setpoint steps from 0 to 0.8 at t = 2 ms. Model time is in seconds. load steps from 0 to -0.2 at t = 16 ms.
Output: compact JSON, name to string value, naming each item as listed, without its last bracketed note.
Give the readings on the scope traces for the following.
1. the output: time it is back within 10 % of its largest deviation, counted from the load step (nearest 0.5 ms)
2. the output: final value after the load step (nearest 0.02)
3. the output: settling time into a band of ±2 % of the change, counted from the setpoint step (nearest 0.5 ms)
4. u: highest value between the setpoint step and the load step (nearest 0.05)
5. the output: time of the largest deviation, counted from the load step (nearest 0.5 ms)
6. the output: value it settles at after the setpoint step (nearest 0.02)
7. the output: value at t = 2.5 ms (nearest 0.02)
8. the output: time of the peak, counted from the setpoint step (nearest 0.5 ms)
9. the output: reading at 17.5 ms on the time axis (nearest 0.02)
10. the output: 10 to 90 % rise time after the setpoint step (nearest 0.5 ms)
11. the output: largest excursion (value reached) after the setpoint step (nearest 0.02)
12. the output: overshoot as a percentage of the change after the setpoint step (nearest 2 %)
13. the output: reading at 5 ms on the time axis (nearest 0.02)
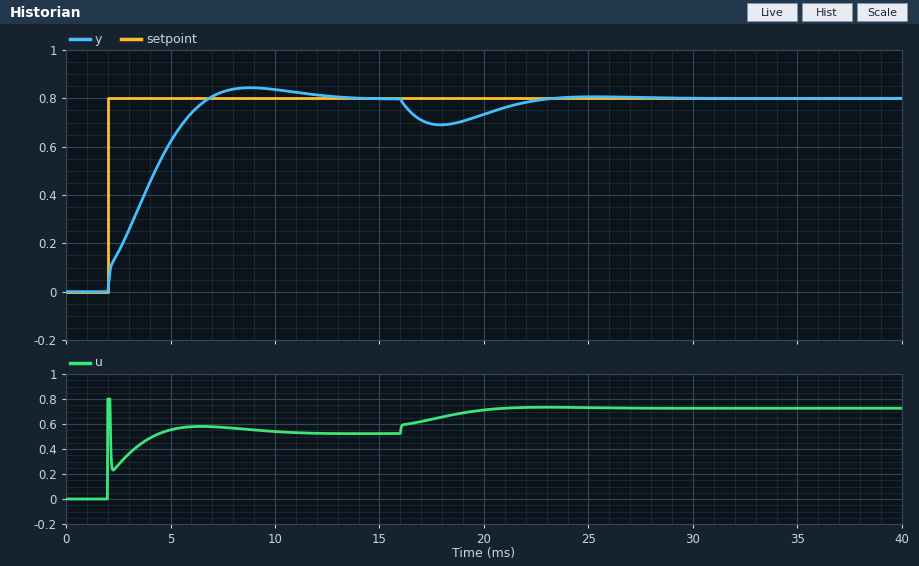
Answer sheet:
{"the output: time it is back within 10 % of its largest deviation, counted from the load step": "6.5 ms", "the output: final value after the load step": "0.80", "the output: settling time into a band of ±2 % of the change, counted from the setpoint step": "10.0 ms", "u: highest value between the setpoint step and the load step": "0.80", "the output: time of the largest deviation, counted from the load step": "2.0 ms", "the output: value it settles at after the setpoint step": "0.80", "the output: value at t = 2.5 ms": "0.16", "the output: time of the peak, counted from the setpoint step": "7.0 ms", "the output: reading at 17.5 ms on the time axis": "0.70", "the output: 10 to 90 % rise time after the setpoint step": "3.5 ms", "the output: largest excursion (value reached) after the setpoint step": "0.84", "the output: overshoot as a percentage of the change after the setpoint step": "6 %", "the output: reading at 5 ms on the time axis": "0.62"}
